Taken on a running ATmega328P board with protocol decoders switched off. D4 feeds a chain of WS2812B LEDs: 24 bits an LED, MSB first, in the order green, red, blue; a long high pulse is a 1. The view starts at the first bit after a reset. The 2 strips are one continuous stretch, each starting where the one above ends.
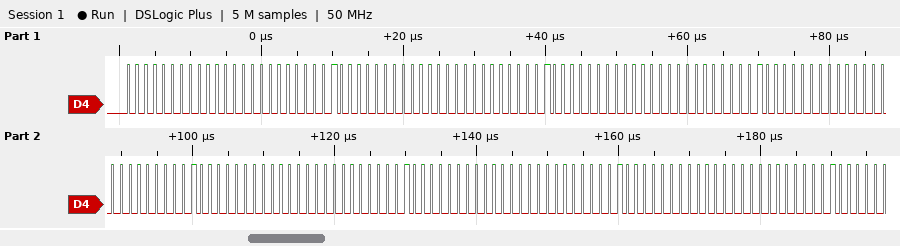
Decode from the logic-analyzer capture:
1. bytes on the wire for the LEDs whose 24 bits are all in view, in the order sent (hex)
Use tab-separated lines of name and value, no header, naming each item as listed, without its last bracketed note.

bytes on the wire for the LEDs whose 24 bits are all in view, in the order sent	00 00 01 00 00 01 00 00 01 00 00 01 00 00 01 00 00 01 00 00 01
